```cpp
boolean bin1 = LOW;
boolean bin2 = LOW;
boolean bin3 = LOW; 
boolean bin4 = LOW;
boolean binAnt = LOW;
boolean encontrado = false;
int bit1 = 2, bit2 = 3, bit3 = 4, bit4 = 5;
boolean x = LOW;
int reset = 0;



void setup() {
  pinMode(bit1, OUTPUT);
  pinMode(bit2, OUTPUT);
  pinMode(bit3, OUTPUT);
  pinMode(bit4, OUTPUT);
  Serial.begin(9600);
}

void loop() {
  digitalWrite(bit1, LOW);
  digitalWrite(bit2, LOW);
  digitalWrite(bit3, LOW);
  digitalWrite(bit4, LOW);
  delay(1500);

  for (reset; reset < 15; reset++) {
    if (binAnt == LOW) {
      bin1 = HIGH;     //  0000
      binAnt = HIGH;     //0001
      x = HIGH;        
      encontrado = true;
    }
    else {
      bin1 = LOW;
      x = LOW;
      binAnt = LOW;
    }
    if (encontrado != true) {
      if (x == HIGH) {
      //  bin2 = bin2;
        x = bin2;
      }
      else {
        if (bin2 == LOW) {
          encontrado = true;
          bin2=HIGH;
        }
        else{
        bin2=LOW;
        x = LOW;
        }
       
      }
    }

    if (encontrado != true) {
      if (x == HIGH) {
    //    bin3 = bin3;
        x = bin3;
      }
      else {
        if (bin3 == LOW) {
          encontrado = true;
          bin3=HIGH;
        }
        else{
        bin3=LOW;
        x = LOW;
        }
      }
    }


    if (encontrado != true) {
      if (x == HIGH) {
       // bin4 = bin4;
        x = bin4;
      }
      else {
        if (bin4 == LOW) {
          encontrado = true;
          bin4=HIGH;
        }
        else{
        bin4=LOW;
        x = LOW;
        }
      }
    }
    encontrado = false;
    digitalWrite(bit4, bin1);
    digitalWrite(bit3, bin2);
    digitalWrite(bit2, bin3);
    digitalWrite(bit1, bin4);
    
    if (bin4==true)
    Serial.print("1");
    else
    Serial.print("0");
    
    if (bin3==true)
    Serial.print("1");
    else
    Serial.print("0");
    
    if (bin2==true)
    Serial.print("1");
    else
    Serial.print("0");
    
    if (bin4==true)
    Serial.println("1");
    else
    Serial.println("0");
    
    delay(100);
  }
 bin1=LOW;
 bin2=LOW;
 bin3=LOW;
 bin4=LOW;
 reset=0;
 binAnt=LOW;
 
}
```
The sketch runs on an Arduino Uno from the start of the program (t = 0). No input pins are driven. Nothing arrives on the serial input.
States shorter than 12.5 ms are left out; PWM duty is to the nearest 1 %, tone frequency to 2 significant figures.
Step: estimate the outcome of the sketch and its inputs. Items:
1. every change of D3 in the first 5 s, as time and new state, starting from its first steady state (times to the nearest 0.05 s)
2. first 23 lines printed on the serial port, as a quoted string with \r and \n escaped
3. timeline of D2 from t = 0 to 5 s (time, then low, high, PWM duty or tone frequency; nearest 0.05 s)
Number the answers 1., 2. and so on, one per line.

1. 0 s low; 1.8 s high; 2.2 s low; 2.6 s high; 3 s low; 4.8 s high
2. "0000\r\n0010\r\n0010\r\n0100\r\n0100\r\n0110\r\n0110\r\n1001\r\n1001\r\n1011\r\n1011\r\n1101\r\n1101\r\n1111\r\n1111\r\n0000\r\n0010\r\n0010\r\n0100\r\n0100\r\n0110\r\n0110\r\n1001\r\n"
3. 0 s low; 2.2 s high; 3 s low
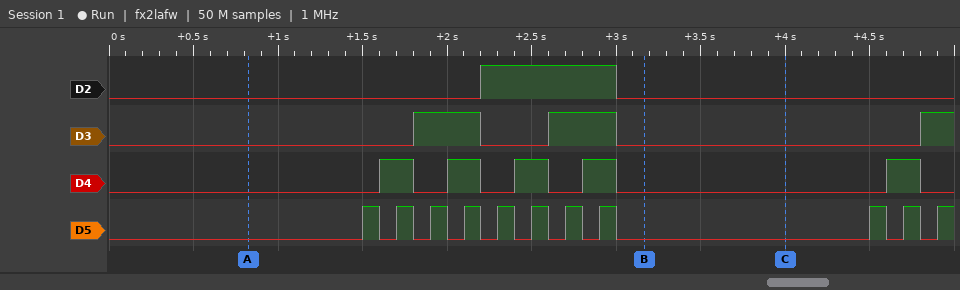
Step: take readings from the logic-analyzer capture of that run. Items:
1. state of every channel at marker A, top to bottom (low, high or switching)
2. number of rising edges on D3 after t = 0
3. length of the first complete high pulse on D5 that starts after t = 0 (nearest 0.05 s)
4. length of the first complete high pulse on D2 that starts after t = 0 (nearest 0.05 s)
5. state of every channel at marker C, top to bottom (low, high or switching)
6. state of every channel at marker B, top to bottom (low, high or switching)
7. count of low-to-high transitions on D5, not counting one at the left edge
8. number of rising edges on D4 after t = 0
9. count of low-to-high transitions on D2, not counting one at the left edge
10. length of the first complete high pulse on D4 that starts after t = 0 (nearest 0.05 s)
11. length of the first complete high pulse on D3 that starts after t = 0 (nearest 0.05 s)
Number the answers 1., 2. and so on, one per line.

1. D2 low, D3 low, D4 low, D5 low
2. 3
3. 0.10 s
4. 0.80 s
5. D2 low, D3 low, D4 low, D5 low
6. D2 low, D3 low, D4 low, D5 low
7. 11
8. 5
9. 1
10. 0.20 s
11. 0.40 s
